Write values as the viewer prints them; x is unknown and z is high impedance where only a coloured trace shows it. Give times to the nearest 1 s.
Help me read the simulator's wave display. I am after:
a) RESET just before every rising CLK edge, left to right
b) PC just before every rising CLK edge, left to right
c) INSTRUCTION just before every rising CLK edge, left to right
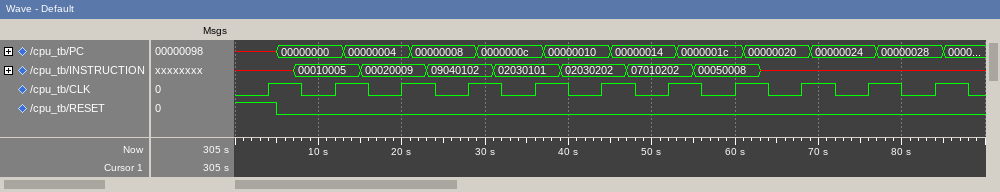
1 0 0 0 0 0 0 0 0 0 0
x, 00000000, 00000004, 00000008, 0000000c, 00000010, 00000014, 0000001c, 00000020, 00000024, 00000028
x, 00010005, 00020009, 09040102, 02030101, 02030202, 07010202, 00050008, x, x, x
